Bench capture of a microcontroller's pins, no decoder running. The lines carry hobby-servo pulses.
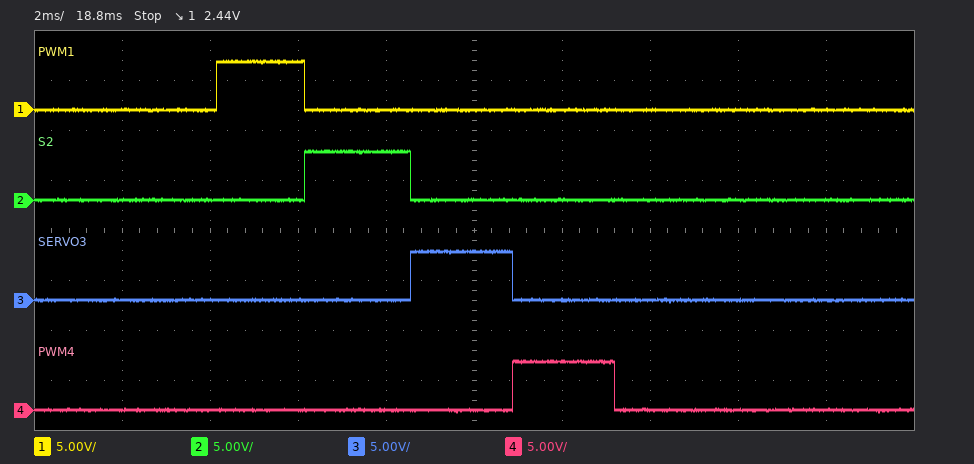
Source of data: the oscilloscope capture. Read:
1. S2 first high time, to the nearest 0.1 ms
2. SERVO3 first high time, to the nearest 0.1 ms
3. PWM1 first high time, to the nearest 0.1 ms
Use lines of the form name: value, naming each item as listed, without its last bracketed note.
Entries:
S2 first high time, to the nearest 0.1 ms: 2.4 ms
SERVO3 first high time, to the nearest 0.1 ms: 2.3 ms
PWM1 first high time, to the nearest 0.1 ms: 2.0 ms
